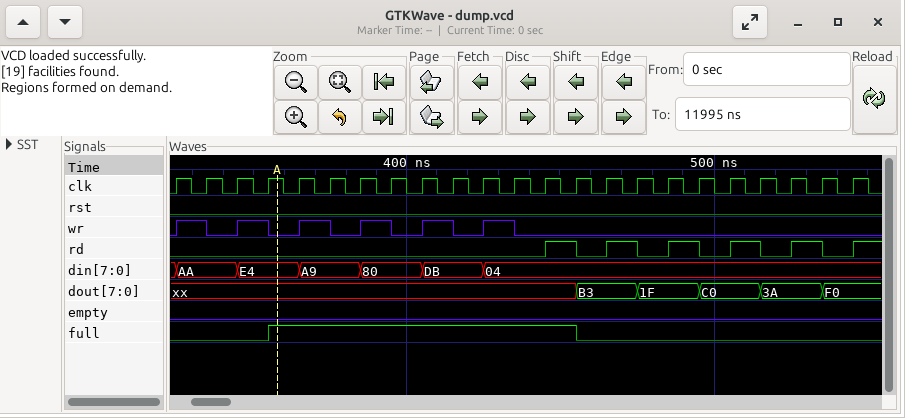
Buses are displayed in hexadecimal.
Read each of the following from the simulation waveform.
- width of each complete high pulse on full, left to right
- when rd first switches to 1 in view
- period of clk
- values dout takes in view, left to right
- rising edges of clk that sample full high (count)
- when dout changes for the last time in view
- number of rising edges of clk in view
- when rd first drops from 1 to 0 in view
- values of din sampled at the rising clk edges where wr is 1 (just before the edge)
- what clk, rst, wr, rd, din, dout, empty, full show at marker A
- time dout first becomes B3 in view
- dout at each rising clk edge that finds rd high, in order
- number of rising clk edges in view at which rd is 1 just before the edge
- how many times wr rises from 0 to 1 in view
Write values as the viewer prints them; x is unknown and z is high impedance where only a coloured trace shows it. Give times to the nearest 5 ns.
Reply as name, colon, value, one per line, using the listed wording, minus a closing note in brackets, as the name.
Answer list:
width of each complete high pulse on full, left to right: 100 ns
when rd first switches to 1 in view: 445 ns
period of clk: 10 ns
values dout takes in view, left to right: xx, B3, 1F, C0, 3A, F0
rising edges of clk that sample full high: 10
when dout changes for the last time in view: 535 ns
number of rising edges of clk in view: 23
when rd first drops from 1 to 0 in view: 455 ns
values of din sampled at the rising clk edges where wr is 1: AA, E4, A9, 80, DB, 04
what clk, rst, wr, rd, din, dout, empty, full show at marker A: clk=1, rst=0, wr=0, rd=0, din=E4, dout=xx, empty=0, full=1
time dout first becomes B3 in view: 455 ns
dout at each rising clk edge that finds rd high, in order: xx, B3, 1F, C0, 3A
number of rising clk edges in view at which rd is 1 just before the edge: 5
how many times wr rises from 0 to 1 in view: 6
